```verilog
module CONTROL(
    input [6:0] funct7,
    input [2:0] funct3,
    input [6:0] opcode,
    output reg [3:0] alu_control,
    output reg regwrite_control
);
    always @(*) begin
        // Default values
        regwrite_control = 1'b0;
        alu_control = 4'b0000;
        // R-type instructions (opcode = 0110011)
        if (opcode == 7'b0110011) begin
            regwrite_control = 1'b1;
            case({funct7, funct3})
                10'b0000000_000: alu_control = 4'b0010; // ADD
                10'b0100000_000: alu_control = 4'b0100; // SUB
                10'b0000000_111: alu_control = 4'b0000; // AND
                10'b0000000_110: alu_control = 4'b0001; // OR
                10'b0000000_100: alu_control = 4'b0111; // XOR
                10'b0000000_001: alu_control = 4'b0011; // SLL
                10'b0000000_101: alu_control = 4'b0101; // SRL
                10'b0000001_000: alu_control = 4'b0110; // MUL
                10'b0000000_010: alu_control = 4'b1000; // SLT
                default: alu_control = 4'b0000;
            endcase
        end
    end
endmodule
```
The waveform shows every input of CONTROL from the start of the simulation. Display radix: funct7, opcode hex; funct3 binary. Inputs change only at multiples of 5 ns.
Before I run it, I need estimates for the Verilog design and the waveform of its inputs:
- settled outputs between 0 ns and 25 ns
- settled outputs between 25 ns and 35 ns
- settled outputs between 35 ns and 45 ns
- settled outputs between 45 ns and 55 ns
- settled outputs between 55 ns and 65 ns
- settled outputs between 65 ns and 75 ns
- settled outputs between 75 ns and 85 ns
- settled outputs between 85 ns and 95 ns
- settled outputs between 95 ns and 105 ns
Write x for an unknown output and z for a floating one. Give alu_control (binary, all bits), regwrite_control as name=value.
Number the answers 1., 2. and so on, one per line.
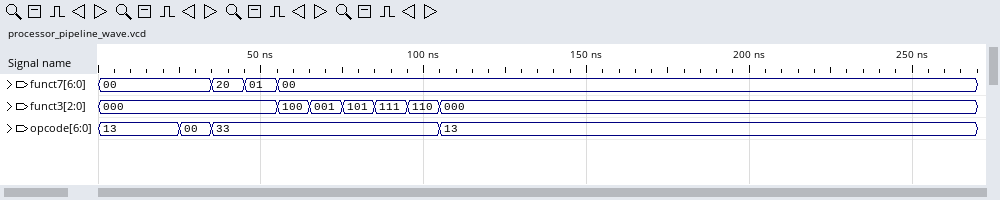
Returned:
1. alu_control=0000, regwrite_control=0
2. alu_control=0000, regwrite_control=0
3. alu_control=0100, regwrite_control=1
4. alu_control=0110, regwrite_control=1
5. alu_control=0111, regwrite_control=1
6. alu_control=0011, regwrite_control=1
7. alu_control=0101, regwrite_control=1
8. alu_control=0000, regwrite_control=1
9. alu_control=0001, regwrite_control=1
